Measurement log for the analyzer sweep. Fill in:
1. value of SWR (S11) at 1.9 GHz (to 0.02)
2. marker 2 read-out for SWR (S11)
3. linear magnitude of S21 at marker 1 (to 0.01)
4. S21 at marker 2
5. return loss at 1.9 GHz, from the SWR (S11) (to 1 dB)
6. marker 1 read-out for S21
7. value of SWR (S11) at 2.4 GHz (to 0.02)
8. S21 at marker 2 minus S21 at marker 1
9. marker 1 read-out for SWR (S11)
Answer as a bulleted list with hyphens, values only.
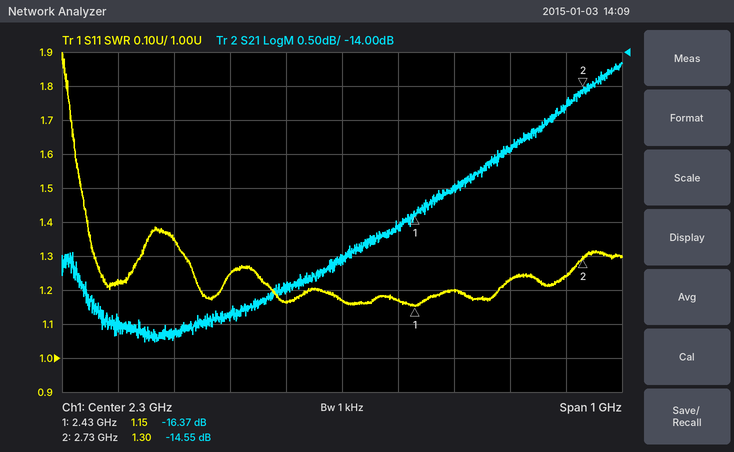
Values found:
- 1.22
- 1.30
- 0.15
- -14.55 dB
- 20 dB
- -16.37 dB
- 1.16
- 1.82 dB
- 1.15
